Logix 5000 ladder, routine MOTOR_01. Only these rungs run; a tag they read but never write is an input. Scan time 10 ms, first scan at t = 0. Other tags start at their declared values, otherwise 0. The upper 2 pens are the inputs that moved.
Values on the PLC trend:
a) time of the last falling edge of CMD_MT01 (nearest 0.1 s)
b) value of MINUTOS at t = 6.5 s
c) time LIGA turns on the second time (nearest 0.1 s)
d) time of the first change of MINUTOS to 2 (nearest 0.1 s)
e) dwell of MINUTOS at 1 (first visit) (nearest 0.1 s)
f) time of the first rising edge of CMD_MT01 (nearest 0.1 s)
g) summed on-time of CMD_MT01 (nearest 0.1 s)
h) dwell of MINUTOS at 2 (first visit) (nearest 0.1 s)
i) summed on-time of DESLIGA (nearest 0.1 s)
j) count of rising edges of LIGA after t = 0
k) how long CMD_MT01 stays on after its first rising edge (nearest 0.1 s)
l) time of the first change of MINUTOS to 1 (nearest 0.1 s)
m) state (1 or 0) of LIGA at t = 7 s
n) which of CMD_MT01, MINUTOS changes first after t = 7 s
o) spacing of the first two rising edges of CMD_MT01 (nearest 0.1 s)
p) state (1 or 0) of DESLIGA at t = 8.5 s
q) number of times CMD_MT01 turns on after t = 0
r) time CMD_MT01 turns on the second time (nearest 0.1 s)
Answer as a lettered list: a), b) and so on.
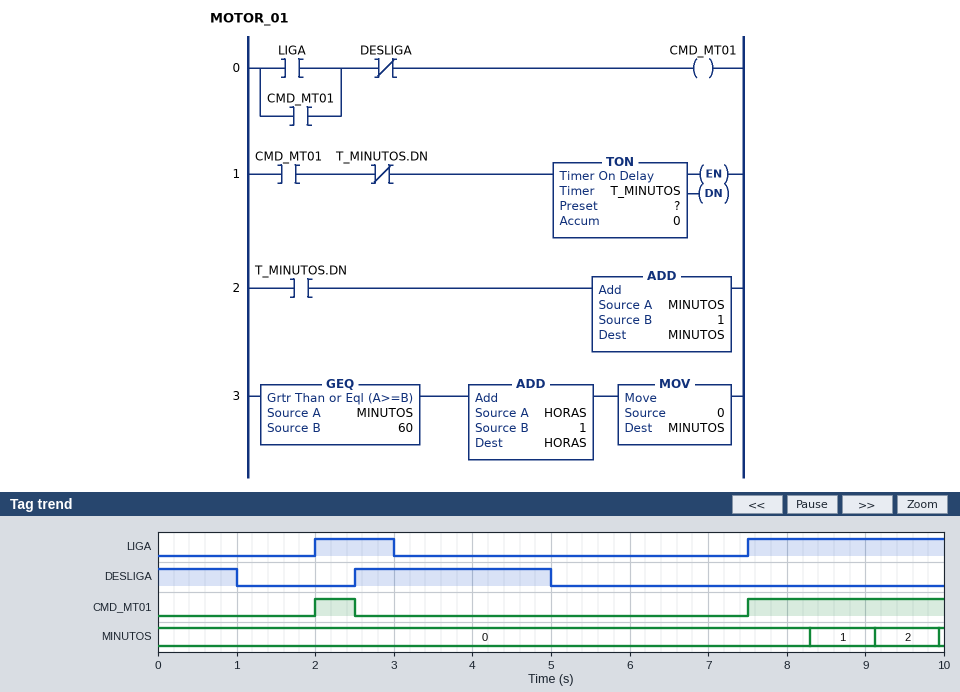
a) 2.5 s
b) 0
c) 7.5 s
d) 9.1 s
e) 0.8 s
f) 2.0 s
g) 3.0 s
h) 0.8 s
i) 3.5 s
j) 2
k) 0.5 s
l) 8.3 s
m) 0
n) CMD_MT01
o) 5.5 s
p) 0
q) 2
r) 7.5 s
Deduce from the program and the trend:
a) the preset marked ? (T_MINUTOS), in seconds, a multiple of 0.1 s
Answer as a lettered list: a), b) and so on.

a) 0.8 s
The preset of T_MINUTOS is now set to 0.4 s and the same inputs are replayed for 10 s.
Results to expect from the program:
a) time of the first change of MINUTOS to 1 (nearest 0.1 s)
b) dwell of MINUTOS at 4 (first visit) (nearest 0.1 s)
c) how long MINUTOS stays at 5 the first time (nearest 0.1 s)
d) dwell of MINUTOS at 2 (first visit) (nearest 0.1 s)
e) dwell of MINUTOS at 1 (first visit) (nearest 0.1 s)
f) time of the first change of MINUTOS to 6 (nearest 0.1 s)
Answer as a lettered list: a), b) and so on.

a) 2.4 s
b) 0.4 s
c) 0.4 s
d) 0.4 s
e) 5.5 s
f) 9.6 s
